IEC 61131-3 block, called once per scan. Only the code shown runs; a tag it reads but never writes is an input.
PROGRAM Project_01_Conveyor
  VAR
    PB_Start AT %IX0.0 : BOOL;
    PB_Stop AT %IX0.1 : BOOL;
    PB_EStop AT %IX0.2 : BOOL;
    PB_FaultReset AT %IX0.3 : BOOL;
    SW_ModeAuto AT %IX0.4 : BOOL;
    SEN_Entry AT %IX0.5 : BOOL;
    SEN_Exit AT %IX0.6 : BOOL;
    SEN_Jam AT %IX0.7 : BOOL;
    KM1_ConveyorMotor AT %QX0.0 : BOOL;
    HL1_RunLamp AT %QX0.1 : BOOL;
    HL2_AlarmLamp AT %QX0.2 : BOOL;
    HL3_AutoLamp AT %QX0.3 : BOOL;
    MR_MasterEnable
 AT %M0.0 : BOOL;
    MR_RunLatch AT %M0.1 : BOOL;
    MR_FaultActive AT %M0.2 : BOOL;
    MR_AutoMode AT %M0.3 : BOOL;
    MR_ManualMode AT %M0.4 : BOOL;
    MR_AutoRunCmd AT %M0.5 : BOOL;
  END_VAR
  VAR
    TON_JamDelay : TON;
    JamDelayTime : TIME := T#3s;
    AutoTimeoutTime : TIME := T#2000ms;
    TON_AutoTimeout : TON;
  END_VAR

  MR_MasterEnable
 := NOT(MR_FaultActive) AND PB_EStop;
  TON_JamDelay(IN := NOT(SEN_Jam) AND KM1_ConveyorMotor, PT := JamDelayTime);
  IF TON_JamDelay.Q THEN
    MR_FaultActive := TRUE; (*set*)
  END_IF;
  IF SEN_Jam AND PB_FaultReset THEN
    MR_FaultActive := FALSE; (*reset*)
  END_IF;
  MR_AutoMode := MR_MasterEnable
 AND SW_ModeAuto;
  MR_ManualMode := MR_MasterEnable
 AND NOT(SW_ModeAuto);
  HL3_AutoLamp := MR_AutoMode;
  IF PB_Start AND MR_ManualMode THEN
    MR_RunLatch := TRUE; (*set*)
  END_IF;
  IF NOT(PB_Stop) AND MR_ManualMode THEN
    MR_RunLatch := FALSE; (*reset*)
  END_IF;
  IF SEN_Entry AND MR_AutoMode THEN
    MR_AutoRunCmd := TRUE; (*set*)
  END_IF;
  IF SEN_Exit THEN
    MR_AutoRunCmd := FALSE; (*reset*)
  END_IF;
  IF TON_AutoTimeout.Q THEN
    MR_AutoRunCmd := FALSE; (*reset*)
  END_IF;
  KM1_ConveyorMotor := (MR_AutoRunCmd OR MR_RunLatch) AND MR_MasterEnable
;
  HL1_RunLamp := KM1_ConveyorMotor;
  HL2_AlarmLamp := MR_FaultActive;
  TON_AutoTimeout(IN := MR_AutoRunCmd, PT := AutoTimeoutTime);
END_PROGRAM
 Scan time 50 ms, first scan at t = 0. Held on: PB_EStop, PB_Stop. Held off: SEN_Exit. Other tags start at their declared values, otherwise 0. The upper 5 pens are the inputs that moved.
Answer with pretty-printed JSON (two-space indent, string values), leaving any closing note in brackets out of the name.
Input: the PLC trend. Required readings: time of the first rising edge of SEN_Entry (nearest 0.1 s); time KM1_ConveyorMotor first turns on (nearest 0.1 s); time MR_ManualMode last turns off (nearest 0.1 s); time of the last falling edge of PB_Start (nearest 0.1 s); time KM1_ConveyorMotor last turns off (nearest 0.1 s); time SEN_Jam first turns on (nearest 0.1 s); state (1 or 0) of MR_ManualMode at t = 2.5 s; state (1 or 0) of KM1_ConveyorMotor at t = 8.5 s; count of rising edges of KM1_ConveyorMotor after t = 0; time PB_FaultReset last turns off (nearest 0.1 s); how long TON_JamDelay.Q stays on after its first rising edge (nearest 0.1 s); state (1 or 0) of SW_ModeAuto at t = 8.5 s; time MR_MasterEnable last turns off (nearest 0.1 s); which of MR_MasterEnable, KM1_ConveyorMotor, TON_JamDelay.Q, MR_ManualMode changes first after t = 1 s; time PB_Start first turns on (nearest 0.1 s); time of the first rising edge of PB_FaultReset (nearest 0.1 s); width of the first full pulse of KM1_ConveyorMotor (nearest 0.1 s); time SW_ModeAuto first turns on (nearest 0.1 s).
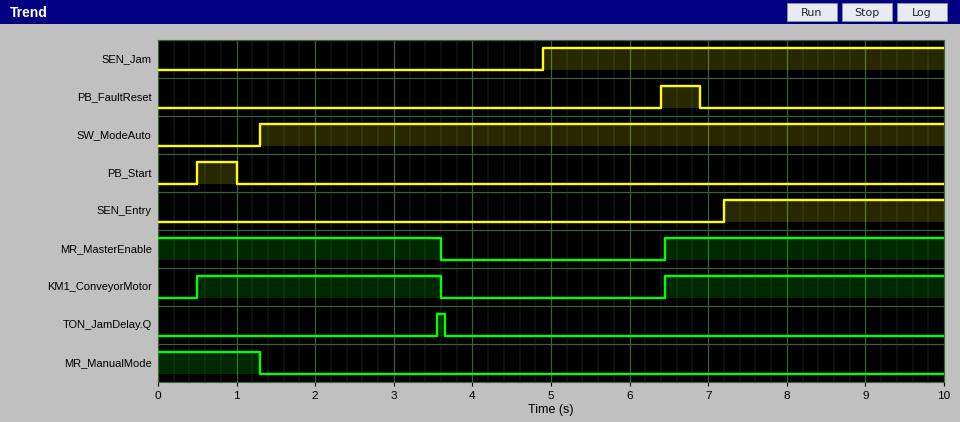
{
  "time of the first rising edge of SEN_Entry": "7.2 s",
  "time KM1_ConveyorMotor first turns on": "0.5 s",
  "time MR_ManualMode last turns off": "1.3 s",
  "time of the last falling edge of PB_Start": "1.0 s",
  "time KM1_ConveyorMotor last turns off": "3.6 s",
  "time SEN_Jam first turns on": "4.9 s",
  "state (1 or 0) of MR_ManualMode at t = 2.5 s": "0",
  "state (1 or 0) of KM1_ConveyorMotor at t = 8.5 s": "1",
  "count of rising edges of KM1_ConveyorMotor after t = 0": "2",
  "time PB_FaultReset last turns off": "6.9 s",
  "how long TON_JamDelay.Q stays on after its first rising edge": "0.1 s",
  "state (1 or 0) of SW_ModeAuto at t = 8.5 s": "1",
  "time MR_MasterEnable last turns off": "3.6 s",
  "which of MR_MasterEnable, KM1_ConveyorMotor, TON_JamDelay.Q, MR_ManualMode changes first after t = 1 s": "MR_ManualMode",
  "time PB_Start first turns on": "0.5 s",
  "time of the first rising edge of PB_FaultReset": "6.4 s",
  "width of the first full pulse of KM1_ConveyorMotor": "3.1 s",
  "time SW_ModeAuto first turns on": "1.3 s"
}
